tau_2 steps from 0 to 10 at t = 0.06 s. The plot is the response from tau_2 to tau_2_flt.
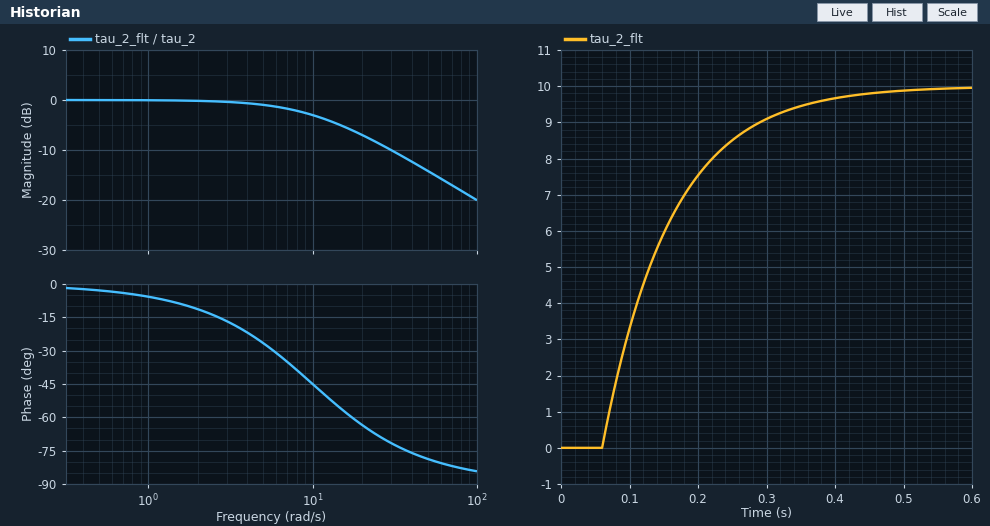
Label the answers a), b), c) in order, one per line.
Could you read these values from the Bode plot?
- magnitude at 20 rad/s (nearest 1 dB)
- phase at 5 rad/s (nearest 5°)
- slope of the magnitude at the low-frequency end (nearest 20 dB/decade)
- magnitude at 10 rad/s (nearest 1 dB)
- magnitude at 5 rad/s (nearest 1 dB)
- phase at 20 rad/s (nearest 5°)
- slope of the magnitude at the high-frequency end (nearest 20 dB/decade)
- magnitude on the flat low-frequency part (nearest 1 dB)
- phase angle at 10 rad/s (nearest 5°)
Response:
a) -7 dB
b) -25°
c) 0 dB/decade
d) -3 dB
e) -1 dB
f) -65°
g) -20 dB/decade
h) 0 dB
i) -45°
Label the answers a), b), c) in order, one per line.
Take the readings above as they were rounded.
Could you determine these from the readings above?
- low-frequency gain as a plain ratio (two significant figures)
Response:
a) 1.0
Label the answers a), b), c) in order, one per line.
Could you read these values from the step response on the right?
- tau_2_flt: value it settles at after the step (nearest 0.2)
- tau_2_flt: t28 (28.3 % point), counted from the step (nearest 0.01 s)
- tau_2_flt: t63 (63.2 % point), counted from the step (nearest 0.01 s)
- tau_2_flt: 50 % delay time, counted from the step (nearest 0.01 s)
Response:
a) 10.0
b) 0.03 s
c) 0.10 s
d) 0.07 s
